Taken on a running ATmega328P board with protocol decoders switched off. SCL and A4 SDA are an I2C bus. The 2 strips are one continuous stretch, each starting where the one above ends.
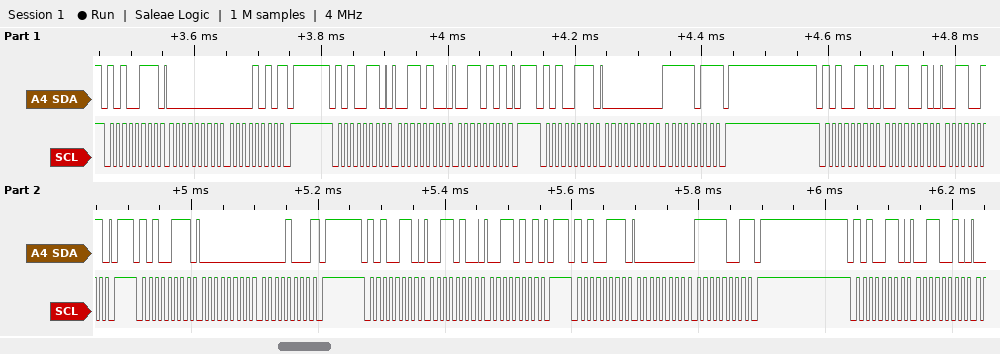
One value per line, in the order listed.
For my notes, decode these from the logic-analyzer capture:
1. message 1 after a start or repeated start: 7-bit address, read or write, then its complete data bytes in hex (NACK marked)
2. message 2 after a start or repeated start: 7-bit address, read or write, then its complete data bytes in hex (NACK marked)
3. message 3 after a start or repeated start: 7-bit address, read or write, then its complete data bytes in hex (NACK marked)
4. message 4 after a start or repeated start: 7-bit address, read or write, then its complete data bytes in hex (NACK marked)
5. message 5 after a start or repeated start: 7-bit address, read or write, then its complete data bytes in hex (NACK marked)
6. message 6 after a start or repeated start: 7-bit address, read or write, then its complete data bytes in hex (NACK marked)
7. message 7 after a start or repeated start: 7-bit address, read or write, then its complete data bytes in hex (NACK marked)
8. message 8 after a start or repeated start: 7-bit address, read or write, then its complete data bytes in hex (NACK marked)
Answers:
0x53 read: 00 0A NACK
0x53 write: 34 35
0x53 read: 00 FB NACK
0x53 write: 32 33
0x53 read: 00 08 NACK
0x53 write: 34 35
0x53 read: 00 F9 NACK
0x53 write: 32
